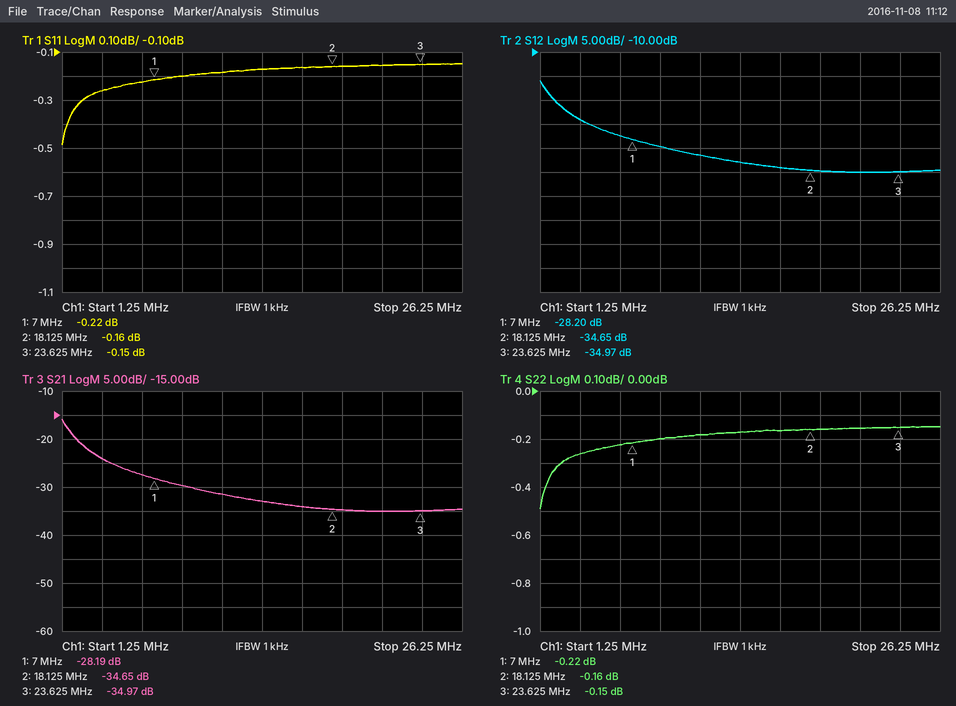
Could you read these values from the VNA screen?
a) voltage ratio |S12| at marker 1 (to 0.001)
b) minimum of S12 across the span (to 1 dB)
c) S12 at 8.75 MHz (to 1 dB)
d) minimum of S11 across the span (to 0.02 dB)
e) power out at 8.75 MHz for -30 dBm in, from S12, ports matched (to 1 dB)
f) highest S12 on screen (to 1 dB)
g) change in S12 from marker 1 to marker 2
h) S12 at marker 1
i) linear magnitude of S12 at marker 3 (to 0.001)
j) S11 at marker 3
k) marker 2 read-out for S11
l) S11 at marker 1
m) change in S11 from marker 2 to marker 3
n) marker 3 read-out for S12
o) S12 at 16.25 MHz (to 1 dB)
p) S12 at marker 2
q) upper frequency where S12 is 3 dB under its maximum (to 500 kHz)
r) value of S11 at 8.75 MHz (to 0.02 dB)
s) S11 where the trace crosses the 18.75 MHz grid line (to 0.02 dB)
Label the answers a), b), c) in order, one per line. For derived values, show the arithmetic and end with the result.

a) 10^(-28.2/20) ≈ 0.039
b) -35 dB
c) -30 dB
d) -0.48 dB
e) -30 dBm + (-30 dB) = -60 dBm
f) -16 dB
g) -34.65 − (-28.2) = -6.45 dB
h) -28.20 dB
i) 10^(-34.97/20) ≈ 0.018
j) -0.15 dB
k) -0.16 dB
l) -0.22 dB
m) -0.15 − (-0.16) = 0.01 dB
n) -34.97 dB
o) -34 dB
p) -34.65 dB
q) 2.0 MHz
r) -0.20 dB
s) -0.16 dB
